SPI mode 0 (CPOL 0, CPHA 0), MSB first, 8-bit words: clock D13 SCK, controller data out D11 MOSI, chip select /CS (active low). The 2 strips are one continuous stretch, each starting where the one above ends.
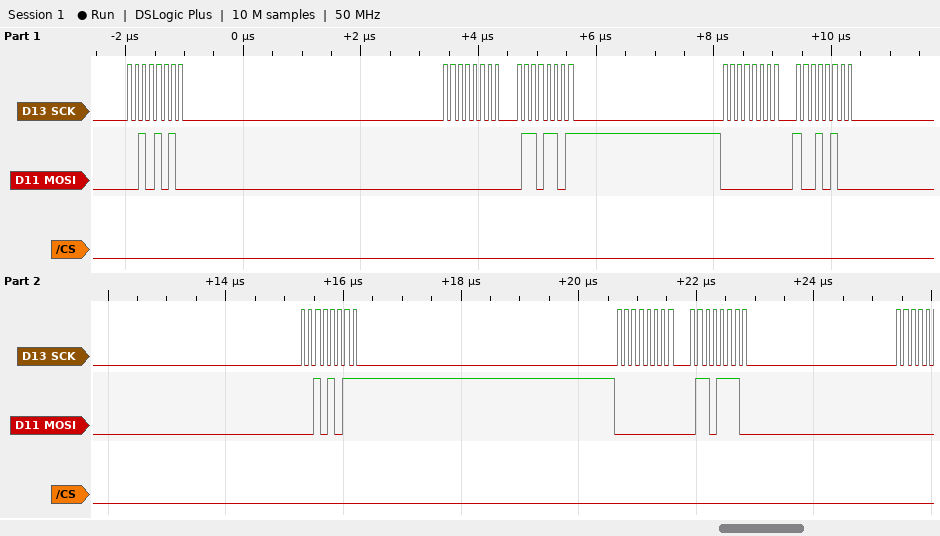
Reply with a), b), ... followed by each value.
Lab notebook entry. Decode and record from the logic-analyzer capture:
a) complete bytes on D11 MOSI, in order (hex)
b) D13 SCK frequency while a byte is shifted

a) 2A 00 6D 00 94 2B 00 6E
b) 8 MHz
